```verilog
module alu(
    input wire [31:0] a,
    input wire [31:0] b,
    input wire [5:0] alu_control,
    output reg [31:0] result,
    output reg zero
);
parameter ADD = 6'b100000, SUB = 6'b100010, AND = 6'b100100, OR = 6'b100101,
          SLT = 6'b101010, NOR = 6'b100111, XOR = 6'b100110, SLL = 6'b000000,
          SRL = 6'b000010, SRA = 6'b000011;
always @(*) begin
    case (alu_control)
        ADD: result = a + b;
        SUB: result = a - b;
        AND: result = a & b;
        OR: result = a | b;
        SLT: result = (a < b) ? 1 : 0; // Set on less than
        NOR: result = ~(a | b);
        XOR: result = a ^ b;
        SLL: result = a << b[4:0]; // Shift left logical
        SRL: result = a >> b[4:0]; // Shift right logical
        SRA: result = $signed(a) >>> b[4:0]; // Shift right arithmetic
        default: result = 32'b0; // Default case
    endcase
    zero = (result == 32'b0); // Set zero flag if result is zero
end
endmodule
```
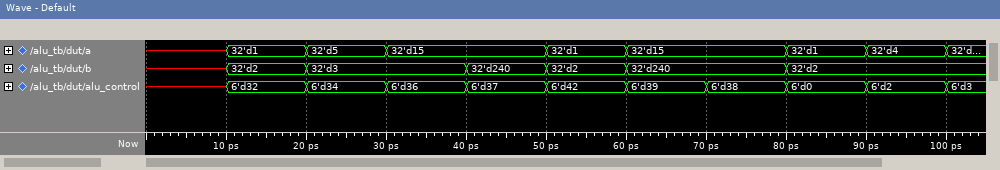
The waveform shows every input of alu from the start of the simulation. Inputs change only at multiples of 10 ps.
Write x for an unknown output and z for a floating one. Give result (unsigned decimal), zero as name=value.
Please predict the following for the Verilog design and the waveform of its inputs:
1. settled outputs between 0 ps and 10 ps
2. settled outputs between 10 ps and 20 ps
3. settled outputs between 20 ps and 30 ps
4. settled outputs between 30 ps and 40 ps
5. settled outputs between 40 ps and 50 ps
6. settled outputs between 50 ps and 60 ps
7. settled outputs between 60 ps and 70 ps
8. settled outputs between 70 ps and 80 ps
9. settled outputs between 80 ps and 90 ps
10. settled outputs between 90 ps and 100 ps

result=x, zero=x
result=3, zero=0
result=2, zero=0
result=3, zero=0
result=255, zero=0
result=1, zero=0
result=4294967040, zero=0
result=255, zero=0
result=4, zero=0
result=1, zero=0
